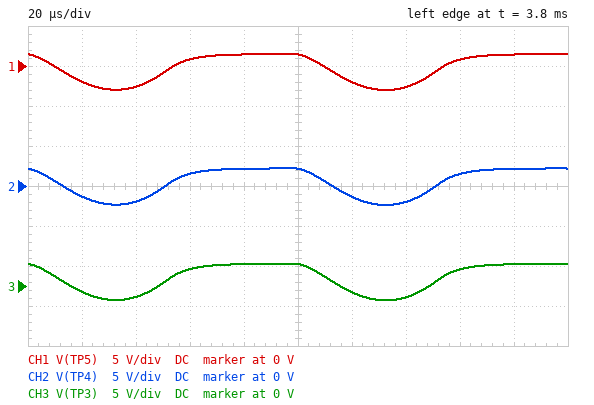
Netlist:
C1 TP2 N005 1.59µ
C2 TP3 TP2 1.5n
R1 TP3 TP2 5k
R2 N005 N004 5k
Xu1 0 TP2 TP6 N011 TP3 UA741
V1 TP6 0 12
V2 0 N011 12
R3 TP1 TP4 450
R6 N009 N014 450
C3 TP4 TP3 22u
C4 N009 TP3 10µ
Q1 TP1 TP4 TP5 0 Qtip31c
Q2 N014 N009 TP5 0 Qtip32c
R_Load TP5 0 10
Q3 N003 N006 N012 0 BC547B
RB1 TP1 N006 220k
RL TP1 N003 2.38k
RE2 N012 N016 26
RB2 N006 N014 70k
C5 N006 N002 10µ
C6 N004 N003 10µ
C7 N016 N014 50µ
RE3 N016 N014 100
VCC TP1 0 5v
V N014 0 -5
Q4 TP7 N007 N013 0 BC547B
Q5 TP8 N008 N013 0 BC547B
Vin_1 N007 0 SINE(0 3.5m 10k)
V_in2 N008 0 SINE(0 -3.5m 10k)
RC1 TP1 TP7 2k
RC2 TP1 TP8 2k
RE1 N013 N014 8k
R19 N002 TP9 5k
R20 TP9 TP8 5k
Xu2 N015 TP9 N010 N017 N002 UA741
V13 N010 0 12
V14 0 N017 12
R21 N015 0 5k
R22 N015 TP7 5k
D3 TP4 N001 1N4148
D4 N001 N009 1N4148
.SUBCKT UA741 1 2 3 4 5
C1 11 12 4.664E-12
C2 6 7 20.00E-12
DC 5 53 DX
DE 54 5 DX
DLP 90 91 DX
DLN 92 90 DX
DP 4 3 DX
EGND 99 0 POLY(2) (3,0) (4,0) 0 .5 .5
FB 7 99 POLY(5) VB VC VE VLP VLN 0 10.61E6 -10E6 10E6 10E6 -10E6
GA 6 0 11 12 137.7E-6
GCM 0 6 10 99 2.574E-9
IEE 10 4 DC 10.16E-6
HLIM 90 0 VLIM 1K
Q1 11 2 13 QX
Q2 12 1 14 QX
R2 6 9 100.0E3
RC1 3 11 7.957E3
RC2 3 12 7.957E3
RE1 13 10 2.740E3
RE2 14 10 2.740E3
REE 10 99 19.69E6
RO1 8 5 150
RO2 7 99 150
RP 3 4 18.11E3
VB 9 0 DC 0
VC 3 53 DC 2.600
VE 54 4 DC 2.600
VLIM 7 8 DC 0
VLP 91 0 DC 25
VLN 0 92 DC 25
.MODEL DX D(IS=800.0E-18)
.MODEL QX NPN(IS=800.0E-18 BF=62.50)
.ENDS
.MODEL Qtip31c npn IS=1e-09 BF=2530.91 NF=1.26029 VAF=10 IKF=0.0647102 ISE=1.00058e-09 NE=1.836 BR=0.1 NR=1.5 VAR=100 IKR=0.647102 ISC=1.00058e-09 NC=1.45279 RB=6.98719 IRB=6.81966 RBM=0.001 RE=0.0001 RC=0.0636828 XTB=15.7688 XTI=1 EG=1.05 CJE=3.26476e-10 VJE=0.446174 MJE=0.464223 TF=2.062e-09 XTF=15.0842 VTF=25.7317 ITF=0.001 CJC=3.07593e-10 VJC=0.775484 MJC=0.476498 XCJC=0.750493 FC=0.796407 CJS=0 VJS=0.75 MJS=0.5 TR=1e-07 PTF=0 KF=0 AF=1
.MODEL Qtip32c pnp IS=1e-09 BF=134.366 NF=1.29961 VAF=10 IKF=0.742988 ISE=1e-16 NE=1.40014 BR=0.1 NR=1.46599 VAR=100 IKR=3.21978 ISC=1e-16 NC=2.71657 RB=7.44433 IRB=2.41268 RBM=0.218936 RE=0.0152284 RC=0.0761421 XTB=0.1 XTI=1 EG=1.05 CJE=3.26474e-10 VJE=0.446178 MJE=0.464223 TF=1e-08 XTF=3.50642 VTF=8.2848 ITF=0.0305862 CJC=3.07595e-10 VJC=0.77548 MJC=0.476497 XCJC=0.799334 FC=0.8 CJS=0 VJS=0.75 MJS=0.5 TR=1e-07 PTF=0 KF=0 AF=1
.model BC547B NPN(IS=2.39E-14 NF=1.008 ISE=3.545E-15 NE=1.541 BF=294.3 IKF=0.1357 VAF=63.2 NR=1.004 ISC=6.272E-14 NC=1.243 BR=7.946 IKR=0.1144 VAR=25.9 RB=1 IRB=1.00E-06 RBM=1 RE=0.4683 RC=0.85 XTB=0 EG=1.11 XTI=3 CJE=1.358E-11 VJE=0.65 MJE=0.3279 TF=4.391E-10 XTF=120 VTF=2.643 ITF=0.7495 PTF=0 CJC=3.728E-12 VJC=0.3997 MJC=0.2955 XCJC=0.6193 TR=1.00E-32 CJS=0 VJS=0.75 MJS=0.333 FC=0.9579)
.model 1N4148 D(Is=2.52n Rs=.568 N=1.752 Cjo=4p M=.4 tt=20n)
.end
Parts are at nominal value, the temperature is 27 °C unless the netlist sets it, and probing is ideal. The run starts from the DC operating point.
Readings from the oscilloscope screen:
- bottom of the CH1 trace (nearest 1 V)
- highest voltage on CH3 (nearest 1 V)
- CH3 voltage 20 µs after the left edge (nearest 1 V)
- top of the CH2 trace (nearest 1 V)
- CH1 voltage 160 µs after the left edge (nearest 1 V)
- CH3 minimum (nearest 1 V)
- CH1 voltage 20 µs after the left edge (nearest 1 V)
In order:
-3 V
3 V
-1 V
2 V
1 V
-2 V
-2 V
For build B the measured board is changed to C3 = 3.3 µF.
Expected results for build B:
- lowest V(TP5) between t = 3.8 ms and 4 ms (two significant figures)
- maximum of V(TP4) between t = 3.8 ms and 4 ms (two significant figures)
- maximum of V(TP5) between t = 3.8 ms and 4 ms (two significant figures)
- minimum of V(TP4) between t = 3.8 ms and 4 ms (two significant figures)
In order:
-3.3 V
1.9 V
1.2 V
-2.6 V
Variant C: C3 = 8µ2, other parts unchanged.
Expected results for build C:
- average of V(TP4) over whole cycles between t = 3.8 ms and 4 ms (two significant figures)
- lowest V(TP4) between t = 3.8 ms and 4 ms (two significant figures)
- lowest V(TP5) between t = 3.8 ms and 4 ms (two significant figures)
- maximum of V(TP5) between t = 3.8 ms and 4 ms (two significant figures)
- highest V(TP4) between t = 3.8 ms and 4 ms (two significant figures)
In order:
290 mV
-2.6 V
-3.2 V
1.3 V
2.0 V
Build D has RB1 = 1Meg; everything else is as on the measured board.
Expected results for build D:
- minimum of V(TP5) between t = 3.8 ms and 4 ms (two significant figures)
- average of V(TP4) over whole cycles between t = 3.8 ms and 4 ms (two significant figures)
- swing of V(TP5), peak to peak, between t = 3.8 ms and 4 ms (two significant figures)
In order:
-3.1 V
470 mV
4.6 V
